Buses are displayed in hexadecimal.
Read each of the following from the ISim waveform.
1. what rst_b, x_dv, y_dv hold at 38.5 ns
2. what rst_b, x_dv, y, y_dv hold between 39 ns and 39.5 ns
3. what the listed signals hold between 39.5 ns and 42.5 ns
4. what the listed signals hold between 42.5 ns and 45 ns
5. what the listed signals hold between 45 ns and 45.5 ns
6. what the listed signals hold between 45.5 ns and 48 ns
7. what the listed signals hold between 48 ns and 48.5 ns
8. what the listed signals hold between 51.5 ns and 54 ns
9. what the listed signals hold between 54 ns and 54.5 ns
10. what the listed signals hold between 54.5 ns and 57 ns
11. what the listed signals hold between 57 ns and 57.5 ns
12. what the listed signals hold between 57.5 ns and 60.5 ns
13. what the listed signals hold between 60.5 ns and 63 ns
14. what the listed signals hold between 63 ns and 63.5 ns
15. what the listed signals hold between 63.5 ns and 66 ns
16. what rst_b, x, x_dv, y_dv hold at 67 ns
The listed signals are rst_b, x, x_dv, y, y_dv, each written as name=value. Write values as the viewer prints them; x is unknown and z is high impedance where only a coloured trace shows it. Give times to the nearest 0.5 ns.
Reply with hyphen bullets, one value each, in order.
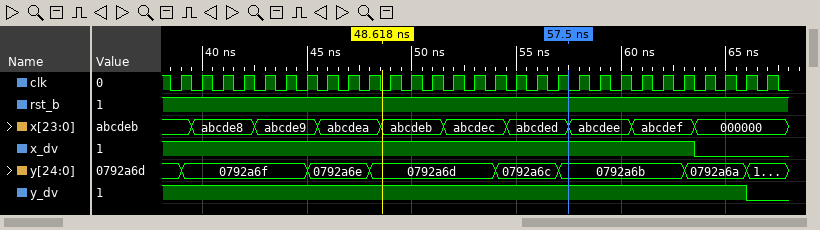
- rst_b=1, x_dv=1, y_dv=1
- rst_b=1, x_dv=1, y=0792a6f, y_dv=1
- rst_b=1, x=abcde8, x_dv=1, y=0792a6f, y_dv=1
- rst_b=1, x=abcde9, x_dv=1, y=0792a6f, y_dv=1
- rst_b=1, x=abcde9, x_dv=1, y=0792a6e, y_dv=1
- rst_b=1, x=abcdea, x_dv=1, y=0792a6e, y_dv=1
- rst_b=1, x=abcdea, x_dv=1, y=0792a6d, y_dv=1
- rst_b=1, x=abcdec, x_dv=1, y=0792a6d, y_dv=1
- rst_b=1, x=abcdec, x_dv=1, y=0792a6c, y_dv=1
- rst_b=1, x=abcded, x_dv=1, y=0792a6c, y_dv=1
- rst_b=1, x=abcded, x_dv=1, y=0792a6b, y_dv=1
- rst_b=1, x=abcdee, x_dv=1, y=0792a6b, y_dv=1
- rst_b=1, x=abcdef, x_dv=1, y=0792a6b, y_dv=1
- rst_b=1, x=abcdef, x_dv=1, y=0792a6a, y_dv=1
- rst_b=1, x=000000, x_dv=0, y=0792a6a, y_dv=1
- rst_b=1, x=000000, x_dv=0, y_dv=0
